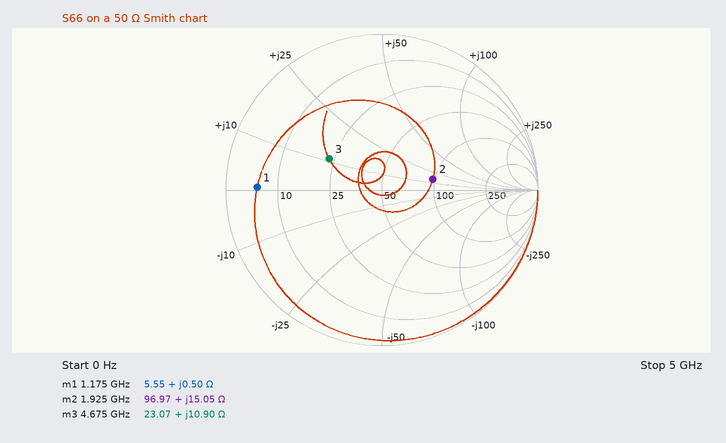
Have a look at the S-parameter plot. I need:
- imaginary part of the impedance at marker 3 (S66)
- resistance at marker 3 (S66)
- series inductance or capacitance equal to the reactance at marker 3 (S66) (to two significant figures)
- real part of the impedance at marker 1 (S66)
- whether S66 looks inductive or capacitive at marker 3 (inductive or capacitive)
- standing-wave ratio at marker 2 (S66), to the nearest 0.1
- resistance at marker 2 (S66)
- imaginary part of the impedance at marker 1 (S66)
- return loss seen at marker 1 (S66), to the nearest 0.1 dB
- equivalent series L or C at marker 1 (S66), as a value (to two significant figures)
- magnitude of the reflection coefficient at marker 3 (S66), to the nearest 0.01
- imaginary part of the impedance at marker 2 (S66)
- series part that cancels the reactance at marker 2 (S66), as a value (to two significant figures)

+10.90 Ω
23.07 Ω
370 pH
5.55 Ω
inductive
2.0
96.97 Ω
+0.50 Ω
1.9 dB
68 pH
0.39
+15.05 Ω
5.5 pF
